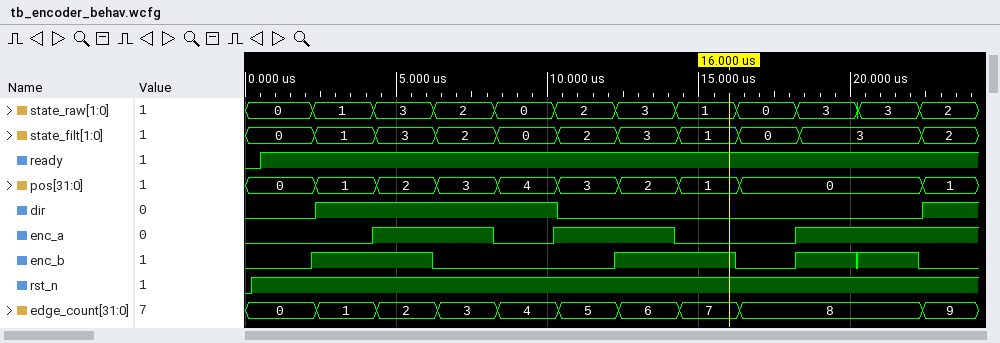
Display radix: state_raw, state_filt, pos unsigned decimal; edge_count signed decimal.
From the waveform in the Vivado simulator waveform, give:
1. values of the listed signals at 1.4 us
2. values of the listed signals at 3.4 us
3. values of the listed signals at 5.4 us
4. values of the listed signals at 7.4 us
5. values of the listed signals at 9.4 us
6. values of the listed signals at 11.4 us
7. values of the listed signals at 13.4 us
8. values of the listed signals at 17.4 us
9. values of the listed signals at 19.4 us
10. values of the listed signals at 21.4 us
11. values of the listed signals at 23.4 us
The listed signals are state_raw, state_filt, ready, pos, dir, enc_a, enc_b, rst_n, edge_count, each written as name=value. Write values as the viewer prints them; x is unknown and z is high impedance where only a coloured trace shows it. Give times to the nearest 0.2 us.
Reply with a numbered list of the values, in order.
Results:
1. state_raw=0, state_filt=0, ready=1, pos=0, dir=0, enc_a=0, enc_b=0, rst_n=1, edge_count=0
2. state_raw=1, state_filt=1, ready=1, pos=1, dir=1, enc_a=0, enc_b=1, rst_n=1, edge_count=1
3. state_raw=3, state_filt=3, ready=1, pos=2, dir=1, enc_a=1, enc_b=1, rst_n=1, edge_count=2
4. state_raw=2, state_filt=2, ready=1, pos=3, dir=1, enc_a=1, enc_b=0, rst_n=1, edge_count=3
5. state_raw=0, state_filt=0, ready=1, pos=4, dir=1, enc_a=0, enc_b=0, rst_n=1, edge_count=4
6. state_raw=2, state_filt=2, ready=1, pos=3, dir=0, enc_a=1, enc_b=0, rst_n=1, edge_count=5
7. state_raw=3, state_filt=3, ready=1, pos=2, dir=0, enc_a=1, enc_b=1, rst_n=1, edge_count=6
8. state_raw=0, state_filt=0, ready=1, pos=0, dir=0, enc_a=0, enc_b=0, rst_n=1, edge_count=8
9. state_raw=3, state_filt=3, ready=1, pos=0, dir=0, enc_a=1, enc_b=1, rst_n=1, edge_count=8
10. state_raw=3, state_filt=3, ready=1, pos=0, dir=0, enc_a=1, enc_b=1, rst_n=1, edge_count=8
11. state_raw=2, state_filt=2, ready=1, pos=1, dir=1, enc_a=1, enc_b=0, rst_n=1, edge_count=9
